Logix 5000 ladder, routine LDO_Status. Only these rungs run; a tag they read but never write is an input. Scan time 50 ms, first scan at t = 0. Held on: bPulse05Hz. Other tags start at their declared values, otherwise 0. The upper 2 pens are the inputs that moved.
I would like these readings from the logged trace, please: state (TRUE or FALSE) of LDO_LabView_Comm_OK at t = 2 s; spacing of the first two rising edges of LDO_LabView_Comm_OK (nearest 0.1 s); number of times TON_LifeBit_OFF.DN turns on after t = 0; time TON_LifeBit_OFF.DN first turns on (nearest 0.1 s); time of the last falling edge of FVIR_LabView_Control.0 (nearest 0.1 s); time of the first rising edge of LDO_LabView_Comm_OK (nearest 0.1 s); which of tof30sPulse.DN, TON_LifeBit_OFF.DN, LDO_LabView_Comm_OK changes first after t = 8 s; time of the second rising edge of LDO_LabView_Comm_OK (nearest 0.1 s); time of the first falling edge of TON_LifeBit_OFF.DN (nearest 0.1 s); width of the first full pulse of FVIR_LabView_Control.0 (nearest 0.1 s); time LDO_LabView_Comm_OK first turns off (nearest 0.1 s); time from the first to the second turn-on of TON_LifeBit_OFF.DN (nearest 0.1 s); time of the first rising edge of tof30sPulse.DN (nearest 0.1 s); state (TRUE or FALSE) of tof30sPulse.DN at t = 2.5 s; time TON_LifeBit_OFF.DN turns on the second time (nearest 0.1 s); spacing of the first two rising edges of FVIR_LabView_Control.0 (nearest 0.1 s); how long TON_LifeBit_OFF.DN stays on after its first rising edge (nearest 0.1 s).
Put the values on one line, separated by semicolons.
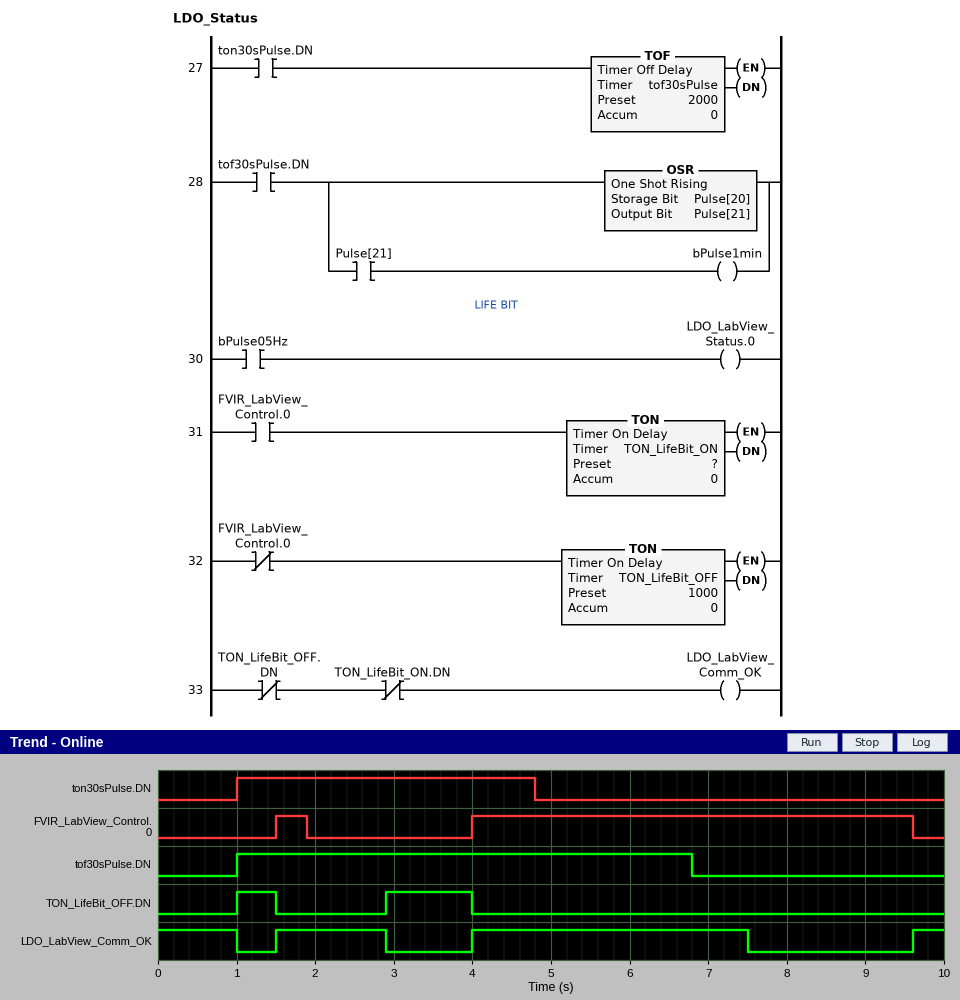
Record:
TRUE; 2.5 s; 2; 1.0 s; 9.6 s; 1.5 s; LDO_LabView_Comm_OK; 4.0 s; 1.5 s; 0.4 s; 1.0 s; 1.9 s; 1.0 s; TRUE; 2.9 s; 2.5 s; 0.5 s
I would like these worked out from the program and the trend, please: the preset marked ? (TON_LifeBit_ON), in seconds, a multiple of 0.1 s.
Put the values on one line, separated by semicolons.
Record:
3.5 s
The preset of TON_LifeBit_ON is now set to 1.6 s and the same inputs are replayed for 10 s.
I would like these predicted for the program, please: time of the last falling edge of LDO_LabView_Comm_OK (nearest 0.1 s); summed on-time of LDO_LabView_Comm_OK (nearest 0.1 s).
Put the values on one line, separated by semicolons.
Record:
5.6 s; 4.4 s
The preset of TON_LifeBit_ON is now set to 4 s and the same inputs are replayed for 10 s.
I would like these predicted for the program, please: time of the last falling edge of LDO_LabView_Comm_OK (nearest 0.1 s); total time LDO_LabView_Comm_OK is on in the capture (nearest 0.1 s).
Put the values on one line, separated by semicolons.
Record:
8.0 s; 6.8 s
